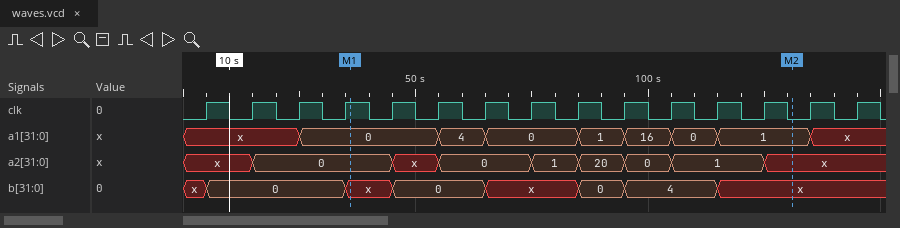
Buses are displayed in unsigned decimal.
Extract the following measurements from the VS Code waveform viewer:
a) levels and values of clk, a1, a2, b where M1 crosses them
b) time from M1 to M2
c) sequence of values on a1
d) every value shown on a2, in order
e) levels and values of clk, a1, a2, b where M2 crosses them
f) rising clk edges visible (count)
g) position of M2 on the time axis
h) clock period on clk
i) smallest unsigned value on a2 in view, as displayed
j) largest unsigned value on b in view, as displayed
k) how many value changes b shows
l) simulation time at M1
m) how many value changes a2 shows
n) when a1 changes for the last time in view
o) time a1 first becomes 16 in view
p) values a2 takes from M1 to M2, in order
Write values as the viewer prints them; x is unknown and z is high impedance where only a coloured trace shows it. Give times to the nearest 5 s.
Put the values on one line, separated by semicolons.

clk=1, a1=0, a2=0, b=x; 95 s; x, 0, 4, 0, 1, 16, 0, 1, x; x, 0, x, 0, 1, 20, 0, 1, x; clk=0, a1=1, a2=x, b=x; 15; 130 s; 10 s; 0; 4; 7; 35 s; 8; 135 s; 95 s; 0, x, 0, 1, 20, 0, 1, x
